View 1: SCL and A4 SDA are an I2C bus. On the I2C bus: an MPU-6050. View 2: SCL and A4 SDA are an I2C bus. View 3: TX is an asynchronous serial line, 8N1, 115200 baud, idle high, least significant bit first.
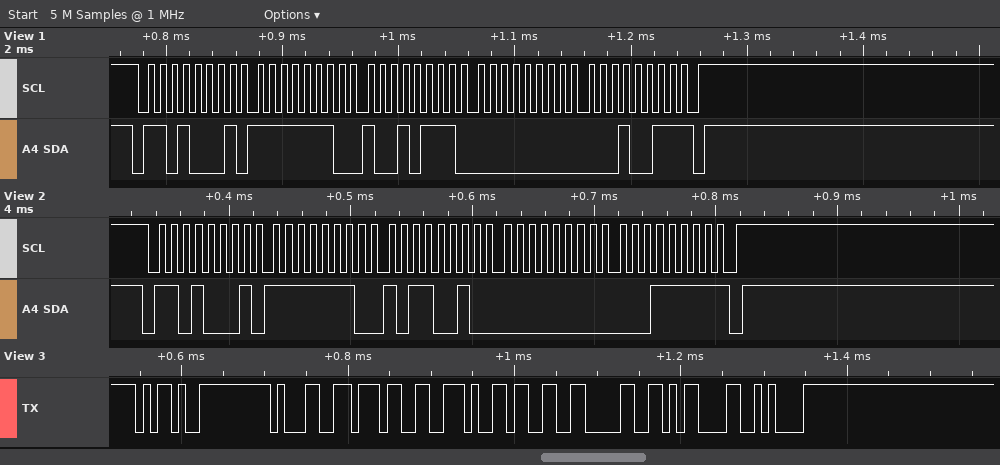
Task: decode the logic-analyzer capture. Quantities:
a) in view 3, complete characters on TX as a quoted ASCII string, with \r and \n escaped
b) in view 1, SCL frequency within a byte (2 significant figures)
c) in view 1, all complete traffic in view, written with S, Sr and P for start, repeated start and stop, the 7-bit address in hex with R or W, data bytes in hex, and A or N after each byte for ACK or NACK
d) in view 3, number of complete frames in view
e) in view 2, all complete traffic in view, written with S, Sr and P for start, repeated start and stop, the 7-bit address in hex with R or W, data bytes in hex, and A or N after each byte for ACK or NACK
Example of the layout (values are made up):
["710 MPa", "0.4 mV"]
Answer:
["\"-17.30\\r\\n\"", "100 kHz", "S 68R A FE A 97 A 00 A 13 N P", "8", "S 68R A FE A B2 A 00 A 1F N P"]
